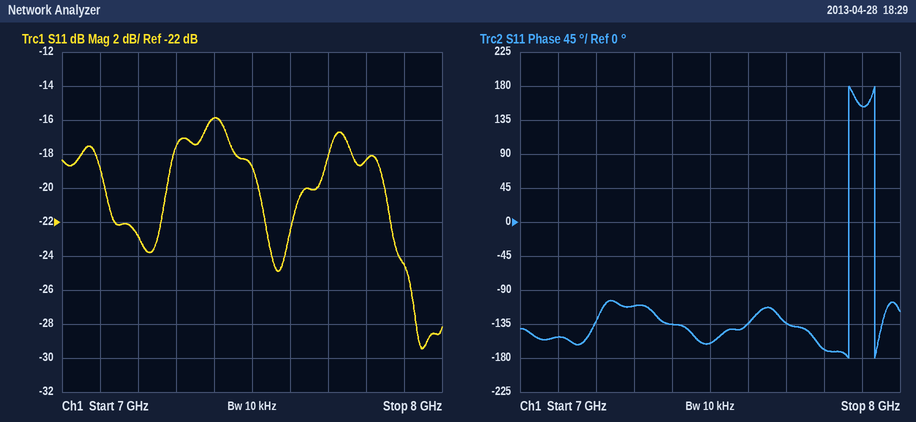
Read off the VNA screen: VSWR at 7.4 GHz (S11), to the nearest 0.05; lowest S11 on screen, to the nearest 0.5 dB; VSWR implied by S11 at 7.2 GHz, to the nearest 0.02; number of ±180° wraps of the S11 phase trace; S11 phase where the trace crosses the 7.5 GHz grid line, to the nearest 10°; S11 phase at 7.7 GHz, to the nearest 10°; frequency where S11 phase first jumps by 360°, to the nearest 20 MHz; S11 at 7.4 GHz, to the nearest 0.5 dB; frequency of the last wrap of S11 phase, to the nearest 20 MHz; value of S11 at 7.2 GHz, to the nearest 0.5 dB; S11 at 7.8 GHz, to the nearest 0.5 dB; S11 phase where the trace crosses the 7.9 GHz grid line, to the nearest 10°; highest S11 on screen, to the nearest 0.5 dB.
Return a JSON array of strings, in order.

["1.40", "-29.5 dB", "1.16", "2", "-160°", "-130°", "7.86 GHz", "-16.0 dB", "7.94 GHz", "-23.0 dB", "-18.5 dB", "150°", "-16.0 dB"]
